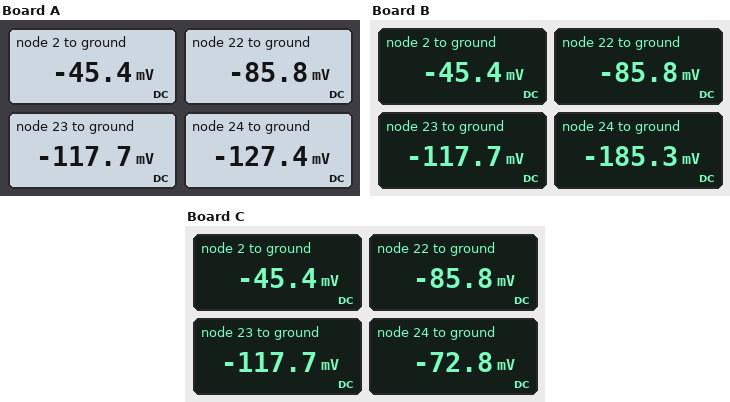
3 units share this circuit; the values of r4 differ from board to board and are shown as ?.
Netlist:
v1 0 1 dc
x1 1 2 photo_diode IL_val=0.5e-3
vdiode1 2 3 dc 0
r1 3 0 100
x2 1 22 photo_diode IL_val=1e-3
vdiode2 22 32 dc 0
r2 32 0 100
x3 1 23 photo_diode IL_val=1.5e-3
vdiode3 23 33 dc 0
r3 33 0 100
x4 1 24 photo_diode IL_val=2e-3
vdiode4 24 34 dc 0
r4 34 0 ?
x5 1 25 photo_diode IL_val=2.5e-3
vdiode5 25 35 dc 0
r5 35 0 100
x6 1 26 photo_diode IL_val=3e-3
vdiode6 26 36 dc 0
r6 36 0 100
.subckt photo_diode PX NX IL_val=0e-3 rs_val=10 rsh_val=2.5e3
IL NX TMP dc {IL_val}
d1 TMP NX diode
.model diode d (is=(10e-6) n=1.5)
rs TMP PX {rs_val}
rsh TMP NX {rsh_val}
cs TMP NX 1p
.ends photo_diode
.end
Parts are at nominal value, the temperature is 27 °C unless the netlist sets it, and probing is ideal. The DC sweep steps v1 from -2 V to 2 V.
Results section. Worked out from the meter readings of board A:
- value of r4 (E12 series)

82 Ω
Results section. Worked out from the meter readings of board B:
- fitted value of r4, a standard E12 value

330 Ω
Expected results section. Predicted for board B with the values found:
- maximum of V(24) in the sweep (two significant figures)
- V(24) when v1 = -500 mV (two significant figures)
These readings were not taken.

1.7 V
270 mV
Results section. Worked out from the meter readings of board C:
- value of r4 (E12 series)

39 Ω
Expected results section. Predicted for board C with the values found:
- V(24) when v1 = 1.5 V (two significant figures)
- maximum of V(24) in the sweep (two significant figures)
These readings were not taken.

-100 mV
1.3 V
